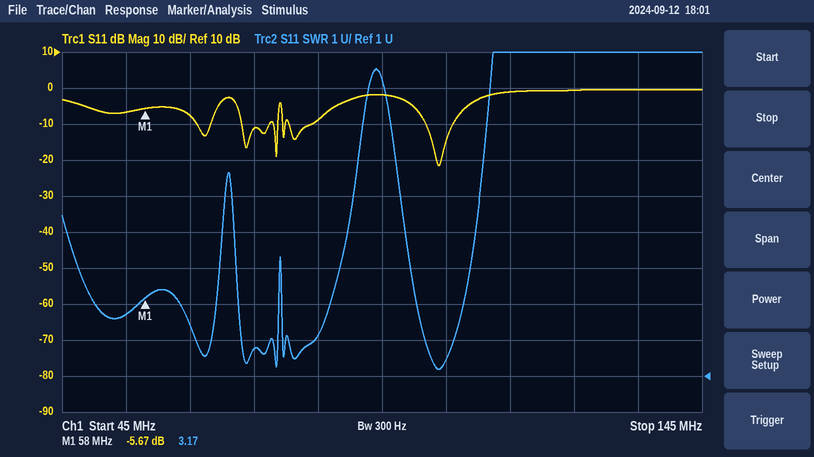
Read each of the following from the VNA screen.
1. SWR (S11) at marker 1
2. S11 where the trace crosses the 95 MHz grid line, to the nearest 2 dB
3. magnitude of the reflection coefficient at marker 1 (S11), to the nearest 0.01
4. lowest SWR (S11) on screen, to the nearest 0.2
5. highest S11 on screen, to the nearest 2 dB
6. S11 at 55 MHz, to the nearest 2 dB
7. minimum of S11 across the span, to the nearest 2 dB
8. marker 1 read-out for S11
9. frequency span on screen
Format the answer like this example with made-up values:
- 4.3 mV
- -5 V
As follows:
- 3.17
- -2 dB
- 0.52
- 1.2
- 0 dB
- -6 dB
- -22 dB
- -5.67 dB
- 100 MHz
